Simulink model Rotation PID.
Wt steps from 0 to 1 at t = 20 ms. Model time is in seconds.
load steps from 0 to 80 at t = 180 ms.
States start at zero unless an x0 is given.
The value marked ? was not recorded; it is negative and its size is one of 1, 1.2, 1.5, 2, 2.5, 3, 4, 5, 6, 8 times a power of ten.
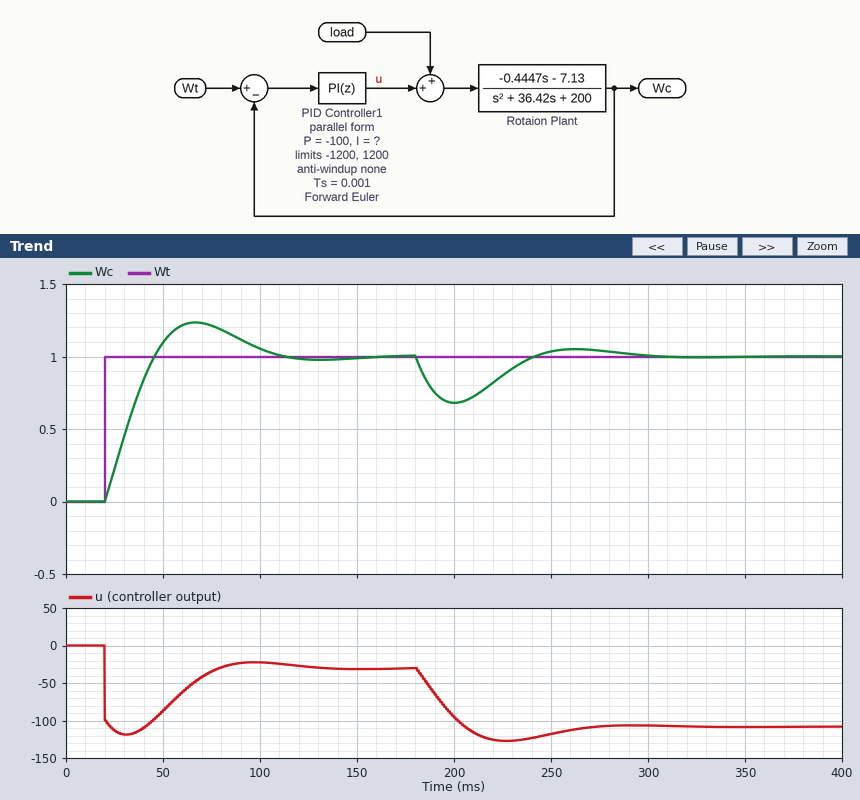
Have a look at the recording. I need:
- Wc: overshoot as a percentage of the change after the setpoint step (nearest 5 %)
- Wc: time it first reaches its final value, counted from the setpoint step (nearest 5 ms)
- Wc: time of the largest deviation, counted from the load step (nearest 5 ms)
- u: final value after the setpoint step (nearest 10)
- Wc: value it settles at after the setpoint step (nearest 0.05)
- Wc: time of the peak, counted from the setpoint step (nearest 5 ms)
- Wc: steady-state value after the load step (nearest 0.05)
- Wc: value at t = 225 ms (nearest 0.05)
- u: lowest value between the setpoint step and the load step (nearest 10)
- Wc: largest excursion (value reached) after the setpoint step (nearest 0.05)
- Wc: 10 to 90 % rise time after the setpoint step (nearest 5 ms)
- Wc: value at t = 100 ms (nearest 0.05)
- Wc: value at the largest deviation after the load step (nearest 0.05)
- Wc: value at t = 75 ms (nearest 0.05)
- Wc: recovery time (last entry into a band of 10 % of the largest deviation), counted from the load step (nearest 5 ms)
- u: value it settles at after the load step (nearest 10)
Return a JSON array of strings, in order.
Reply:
["25 %", "25 ms", "20 ms", "-30", "1.00", "45 ms", "1.00", "0.85", "-120", "1.25", "20 ms", "1.05", "0.70", "1.20", "100 ms", "-110"]
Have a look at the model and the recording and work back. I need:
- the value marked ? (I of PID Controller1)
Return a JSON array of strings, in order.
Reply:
["-8000"]
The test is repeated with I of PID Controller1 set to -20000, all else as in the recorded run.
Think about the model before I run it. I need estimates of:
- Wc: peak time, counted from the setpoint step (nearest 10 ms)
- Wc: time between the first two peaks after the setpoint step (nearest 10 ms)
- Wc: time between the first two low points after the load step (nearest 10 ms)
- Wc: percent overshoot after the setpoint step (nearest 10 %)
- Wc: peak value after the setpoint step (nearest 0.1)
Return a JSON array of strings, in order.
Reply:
["30 ms", "70 ms", "70 ms", "40 %", "1.4"]
